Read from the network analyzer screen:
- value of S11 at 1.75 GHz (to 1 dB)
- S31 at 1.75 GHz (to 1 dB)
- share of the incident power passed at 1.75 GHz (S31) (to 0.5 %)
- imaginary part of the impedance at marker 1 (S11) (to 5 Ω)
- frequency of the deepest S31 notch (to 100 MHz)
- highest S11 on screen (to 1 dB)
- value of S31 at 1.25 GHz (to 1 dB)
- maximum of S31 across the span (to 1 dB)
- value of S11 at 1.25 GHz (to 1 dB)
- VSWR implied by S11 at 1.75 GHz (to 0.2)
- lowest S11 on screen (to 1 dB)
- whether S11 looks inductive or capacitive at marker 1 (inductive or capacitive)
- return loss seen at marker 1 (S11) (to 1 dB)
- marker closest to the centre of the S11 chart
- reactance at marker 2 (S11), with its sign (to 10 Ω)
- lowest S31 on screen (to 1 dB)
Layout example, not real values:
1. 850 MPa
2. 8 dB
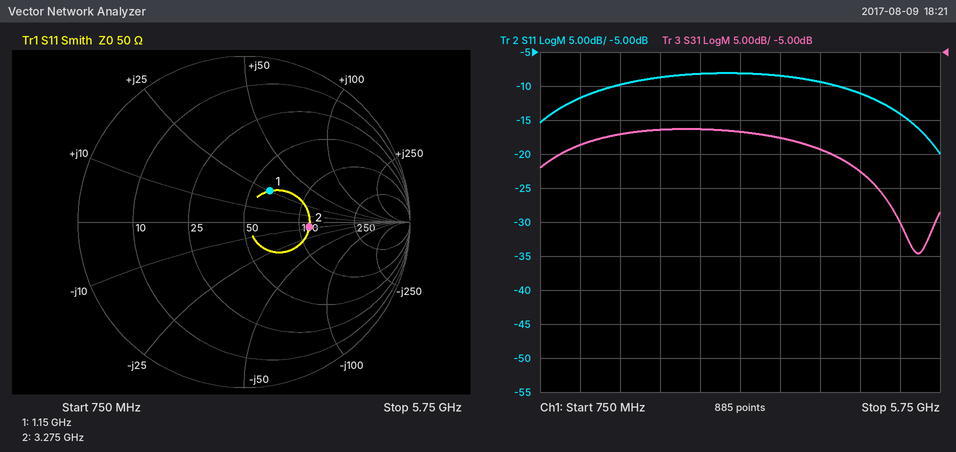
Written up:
1. -10 dB
2. -17 dB
3. 2.0 %
4. +25 Ω
5. 5.5 GHz
6. -8 dB
7. -19 dB
8. -16 dB
9. -12 dB
10. 2.0
11. -20 dB
12. inductive
13. 12 dB
14. marker 1
15. -10 Ω
16. -35 dB
